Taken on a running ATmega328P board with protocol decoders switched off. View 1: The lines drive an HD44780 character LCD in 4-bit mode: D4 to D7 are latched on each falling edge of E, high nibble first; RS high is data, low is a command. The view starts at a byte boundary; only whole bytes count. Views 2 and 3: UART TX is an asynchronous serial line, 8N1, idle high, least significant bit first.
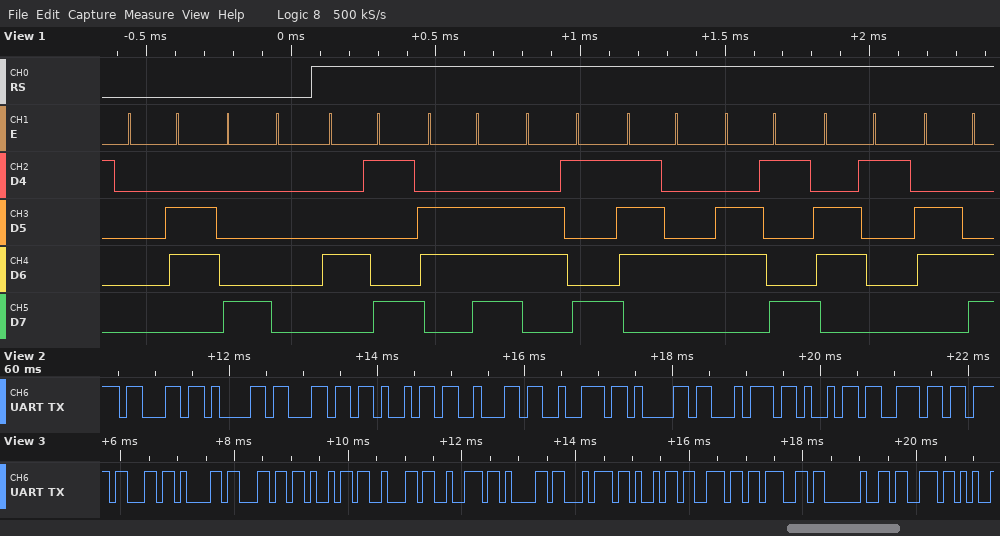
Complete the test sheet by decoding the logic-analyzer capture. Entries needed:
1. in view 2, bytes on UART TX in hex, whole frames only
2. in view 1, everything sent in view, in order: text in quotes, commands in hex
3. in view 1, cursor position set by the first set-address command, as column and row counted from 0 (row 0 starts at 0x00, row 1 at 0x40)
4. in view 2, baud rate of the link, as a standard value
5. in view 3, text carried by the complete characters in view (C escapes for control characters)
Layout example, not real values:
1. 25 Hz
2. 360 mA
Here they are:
1. 63 61 6C 69 62 72 61 74 69 6E
2. 0x06 0x80 "Initial"
3. column 0, row 0
4. 9600 baud
5. "calibrating s"
